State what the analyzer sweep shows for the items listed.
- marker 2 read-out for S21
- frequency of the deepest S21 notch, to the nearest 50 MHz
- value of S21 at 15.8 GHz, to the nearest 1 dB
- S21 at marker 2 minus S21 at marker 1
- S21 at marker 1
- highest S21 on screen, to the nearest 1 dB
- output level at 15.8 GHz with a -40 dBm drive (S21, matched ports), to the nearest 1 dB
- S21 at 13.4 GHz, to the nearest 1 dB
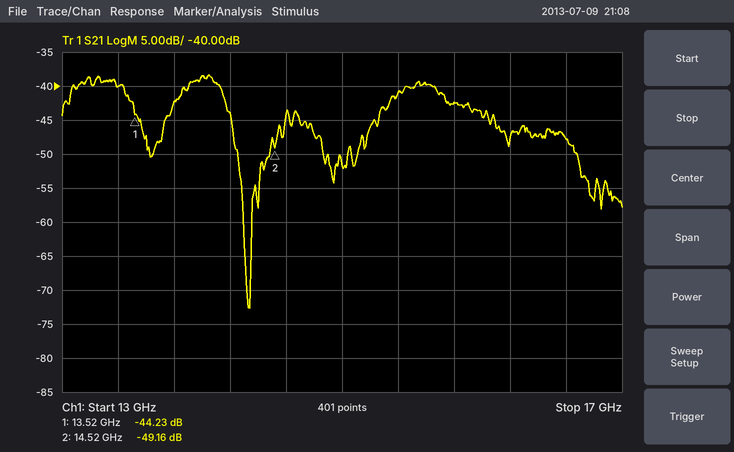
-49.16 dB
14.35 GHz
-42 dB
-4.93 dB
-44.23 dB
-38 dB
-82 dBm
-40 dB
